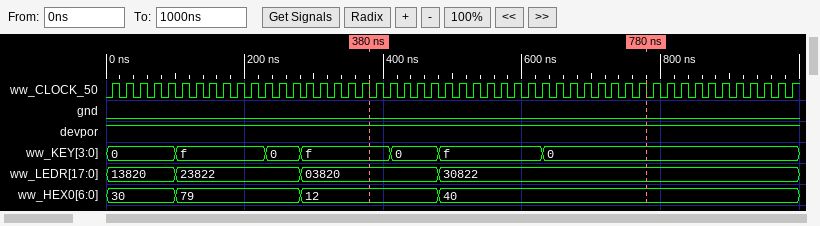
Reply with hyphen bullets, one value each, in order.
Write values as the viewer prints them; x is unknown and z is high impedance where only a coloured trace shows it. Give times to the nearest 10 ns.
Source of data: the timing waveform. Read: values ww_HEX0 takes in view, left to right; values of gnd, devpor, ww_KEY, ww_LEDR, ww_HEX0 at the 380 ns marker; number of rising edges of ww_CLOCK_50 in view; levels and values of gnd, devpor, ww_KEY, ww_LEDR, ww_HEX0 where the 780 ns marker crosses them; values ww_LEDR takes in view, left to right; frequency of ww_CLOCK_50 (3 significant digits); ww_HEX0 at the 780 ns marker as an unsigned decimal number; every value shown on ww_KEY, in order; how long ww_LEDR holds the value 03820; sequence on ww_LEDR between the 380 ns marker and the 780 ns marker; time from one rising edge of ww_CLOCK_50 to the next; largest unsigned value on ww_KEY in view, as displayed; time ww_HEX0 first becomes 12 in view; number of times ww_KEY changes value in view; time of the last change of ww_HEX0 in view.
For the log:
- 30, 79, 12, 40
- gnd=0, devpor=1, ww_KEY=f, ww_LEDR=03820, ww_HEX0=12
- 50
- gnd=0, devpor=1, ww_KEY=0, ww_LEDR=30822, ww_HEX0=40
- 13820, 23822, 03820, 30822
- 50.0 MHz
- 64
- 0, f, 0, f, 0, f, 0
- 200 ns
- 03820, 30822
- 20 ns
- f
- 280 ns
- 6
- 480 ns
